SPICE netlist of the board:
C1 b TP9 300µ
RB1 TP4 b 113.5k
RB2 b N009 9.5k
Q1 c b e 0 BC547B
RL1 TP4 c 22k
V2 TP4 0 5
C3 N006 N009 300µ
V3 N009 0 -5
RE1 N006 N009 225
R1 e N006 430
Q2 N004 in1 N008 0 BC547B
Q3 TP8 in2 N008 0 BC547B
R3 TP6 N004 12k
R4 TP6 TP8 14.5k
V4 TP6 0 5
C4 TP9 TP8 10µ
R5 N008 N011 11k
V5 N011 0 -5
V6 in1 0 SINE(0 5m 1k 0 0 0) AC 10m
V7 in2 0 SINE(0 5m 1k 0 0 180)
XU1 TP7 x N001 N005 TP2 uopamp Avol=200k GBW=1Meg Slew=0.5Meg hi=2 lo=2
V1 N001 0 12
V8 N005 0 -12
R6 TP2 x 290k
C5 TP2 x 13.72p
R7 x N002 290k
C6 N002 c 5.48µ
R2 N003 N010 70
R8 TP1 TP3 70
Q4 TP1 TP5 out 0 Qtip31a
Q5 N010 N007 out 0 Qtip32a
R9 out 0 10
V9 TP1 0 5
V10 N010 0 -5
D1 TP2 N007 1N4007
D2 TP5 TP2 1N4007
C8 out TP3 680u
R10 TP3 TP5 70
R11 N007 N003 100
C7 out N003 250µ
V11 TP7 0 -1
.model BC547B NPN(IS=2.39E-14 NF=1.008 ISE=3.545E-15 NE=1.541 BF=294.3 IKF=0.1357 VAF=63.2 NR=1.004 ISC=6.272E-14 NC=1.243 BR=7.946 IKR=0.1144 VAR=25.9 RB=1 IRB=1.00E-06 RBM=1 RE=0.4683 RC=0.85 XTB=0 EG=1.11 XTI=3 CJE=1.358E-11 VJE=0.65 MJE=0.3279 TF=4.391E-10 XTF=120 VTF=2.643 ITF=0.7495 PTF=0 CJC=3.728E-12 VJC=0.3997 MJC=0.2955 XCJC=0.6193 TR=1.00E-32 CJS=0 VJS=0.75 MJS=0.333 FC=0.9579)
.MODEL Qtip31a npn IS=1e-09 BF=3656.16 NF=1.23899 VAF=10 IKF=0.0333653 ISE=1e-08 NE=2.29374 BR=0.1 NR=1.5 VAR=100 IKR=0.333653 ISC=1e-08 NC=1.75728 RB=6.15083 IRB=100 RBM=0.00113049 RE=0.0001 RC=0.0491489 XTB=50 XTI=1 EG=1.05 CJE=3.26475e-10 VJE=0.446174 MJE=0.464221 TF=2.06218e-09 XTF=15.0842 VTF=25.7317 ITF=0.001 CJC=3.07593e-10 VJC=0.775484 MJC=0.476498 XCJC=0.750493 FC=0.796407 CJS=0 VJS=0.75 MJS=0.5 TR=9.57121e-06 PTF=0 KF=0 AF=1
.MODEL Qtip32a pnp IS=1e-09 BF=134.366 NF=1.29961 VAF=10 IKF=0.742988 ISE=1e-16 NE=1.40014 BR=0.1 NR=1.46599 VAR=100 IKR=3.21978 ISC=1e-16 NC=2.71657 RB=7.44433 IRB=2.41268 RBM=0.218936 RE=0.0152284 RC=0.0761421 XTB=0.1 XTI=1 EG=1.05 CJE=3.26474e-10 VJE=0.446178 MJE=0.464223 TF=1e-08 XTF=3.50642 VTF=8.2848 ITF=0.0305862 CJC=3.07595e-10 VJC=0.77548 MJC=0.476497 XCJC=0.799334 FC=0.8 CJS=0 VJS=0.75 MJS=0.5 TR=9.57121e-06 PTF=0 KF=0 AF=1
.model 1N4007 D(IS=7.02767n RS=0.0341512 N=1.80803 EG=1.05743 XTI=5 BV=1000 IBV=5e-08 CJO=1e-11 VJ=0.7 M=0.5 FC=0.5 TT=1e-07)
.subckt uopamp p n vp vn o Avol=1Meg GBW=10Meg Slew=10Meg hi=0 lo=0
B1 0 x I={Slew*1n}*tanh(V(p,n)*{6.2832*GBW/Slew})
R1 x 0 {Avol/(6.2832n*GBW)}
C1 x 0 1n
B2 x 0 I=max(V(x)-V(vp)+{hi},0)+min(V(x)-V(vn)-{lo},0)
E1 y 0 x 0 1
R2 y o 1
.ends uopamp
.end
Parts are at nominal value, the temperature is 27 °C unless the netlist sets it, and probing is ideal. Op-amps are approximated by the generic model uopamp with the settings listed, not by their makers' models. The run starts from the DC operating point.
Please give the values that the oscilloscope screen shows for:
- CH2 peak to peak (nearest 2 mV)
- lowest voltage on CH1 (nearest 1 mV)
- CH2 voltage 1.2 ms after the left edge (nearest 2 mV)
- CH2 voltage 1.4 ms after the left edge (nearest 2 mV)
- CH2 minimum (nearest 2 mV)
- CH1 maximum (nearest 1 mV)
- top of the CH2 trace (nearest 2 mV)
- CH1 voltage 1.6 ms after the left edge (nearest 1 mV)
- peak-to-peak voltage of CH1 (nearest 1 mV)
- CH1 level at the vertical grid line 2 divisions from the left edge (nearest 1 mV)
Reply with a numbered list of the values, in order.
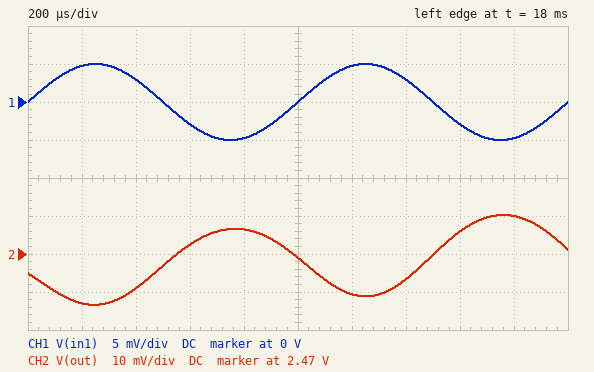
1. 24 mV
2. -5 mV
3. 2.460 V
4. 2.464 V
5. 2.456 V
6. 5 mV
7. 2.480 V
8. -3 mV
9. 10 mV
10. 3 mV
